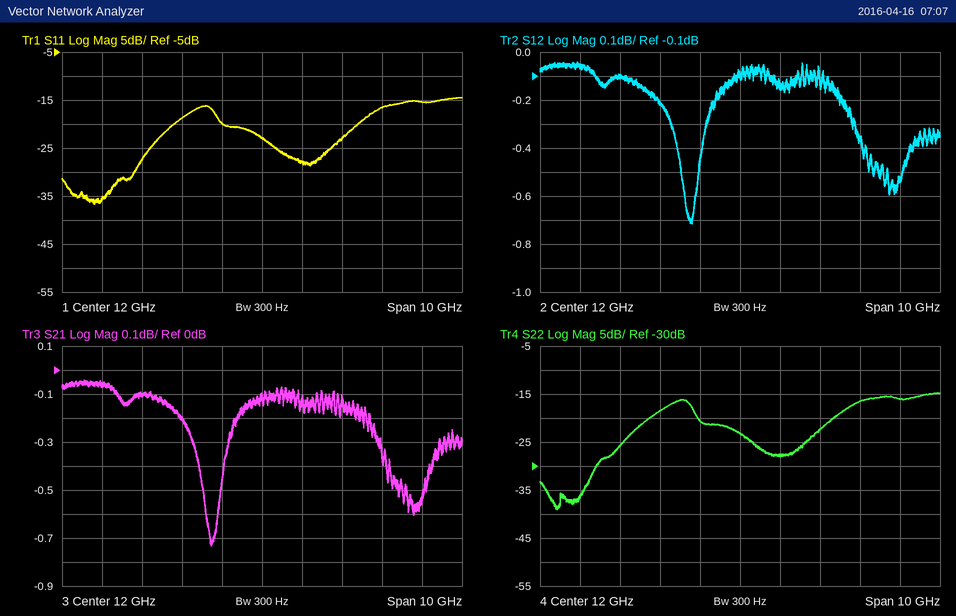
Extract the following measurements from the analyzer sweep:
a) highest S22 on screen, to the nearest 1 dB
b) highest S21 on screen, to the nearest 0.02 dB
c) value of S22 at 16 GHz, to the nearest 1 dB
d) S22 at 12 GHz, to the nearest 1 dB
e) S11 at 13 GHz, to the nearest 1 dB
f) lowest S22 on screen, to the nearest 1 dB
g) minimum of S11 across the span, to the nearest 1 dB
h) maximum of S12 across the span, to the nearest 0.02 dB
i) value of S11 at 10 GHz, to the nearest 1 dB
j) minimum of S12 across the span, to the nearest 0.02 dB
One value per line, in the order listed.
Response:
-15 dB
-0.04 dB
-16 dB
-23 dB
-28 dB
-39 dB
-37 dB
-0.04 dB
-19 dB
-0.72 dB
